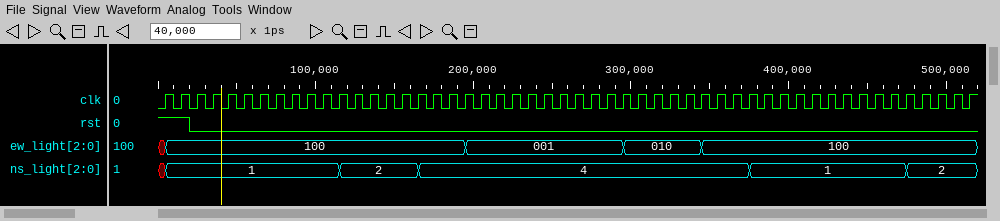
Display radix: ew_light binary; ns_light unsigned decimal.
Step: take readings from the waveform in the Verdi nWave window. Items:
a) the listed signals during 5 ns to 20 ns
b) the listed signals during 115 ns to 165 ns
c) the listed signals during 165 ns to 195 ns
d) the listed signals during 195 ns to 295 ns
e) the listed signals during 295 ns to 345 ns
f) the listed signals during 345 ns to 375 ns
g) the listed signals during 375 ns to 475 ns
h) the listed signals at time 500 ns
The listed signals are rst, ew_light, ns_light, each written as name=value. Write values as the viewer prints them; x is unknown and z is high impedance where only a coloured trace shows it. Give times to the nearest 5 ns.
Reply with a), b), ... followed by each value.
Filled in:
a) rst=1, ew_light=100, ns_light=1
b) rst=0, ew_light=100, ns_light=2
c) rst=0, ew_light=100, ns_light=4
d) rst=0, ew_light=001, ns_light=4
e) rst=0, ew_light=010, ns_light=4
f) rst=0, ew_light=100, ns_light=4
g) rst=0, ew_light=100, ns_light=1
h) rst=0, ew_light=100, ns_light=2
